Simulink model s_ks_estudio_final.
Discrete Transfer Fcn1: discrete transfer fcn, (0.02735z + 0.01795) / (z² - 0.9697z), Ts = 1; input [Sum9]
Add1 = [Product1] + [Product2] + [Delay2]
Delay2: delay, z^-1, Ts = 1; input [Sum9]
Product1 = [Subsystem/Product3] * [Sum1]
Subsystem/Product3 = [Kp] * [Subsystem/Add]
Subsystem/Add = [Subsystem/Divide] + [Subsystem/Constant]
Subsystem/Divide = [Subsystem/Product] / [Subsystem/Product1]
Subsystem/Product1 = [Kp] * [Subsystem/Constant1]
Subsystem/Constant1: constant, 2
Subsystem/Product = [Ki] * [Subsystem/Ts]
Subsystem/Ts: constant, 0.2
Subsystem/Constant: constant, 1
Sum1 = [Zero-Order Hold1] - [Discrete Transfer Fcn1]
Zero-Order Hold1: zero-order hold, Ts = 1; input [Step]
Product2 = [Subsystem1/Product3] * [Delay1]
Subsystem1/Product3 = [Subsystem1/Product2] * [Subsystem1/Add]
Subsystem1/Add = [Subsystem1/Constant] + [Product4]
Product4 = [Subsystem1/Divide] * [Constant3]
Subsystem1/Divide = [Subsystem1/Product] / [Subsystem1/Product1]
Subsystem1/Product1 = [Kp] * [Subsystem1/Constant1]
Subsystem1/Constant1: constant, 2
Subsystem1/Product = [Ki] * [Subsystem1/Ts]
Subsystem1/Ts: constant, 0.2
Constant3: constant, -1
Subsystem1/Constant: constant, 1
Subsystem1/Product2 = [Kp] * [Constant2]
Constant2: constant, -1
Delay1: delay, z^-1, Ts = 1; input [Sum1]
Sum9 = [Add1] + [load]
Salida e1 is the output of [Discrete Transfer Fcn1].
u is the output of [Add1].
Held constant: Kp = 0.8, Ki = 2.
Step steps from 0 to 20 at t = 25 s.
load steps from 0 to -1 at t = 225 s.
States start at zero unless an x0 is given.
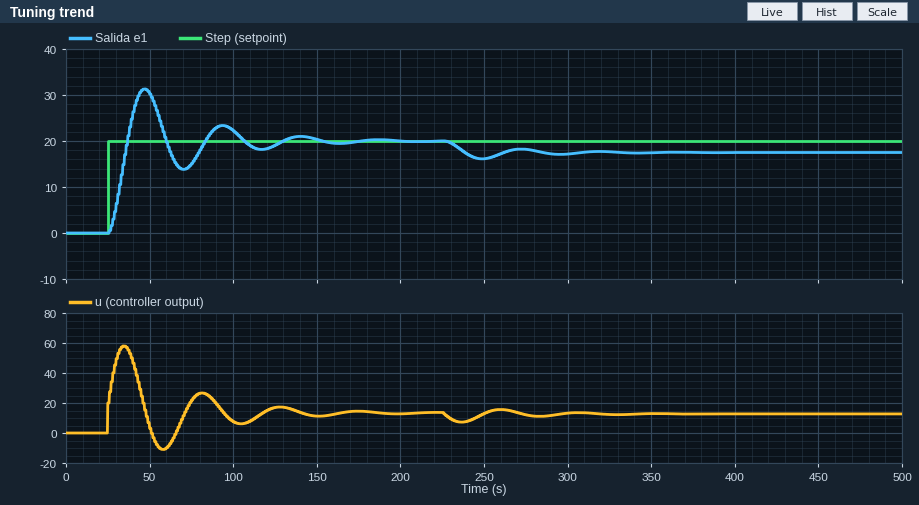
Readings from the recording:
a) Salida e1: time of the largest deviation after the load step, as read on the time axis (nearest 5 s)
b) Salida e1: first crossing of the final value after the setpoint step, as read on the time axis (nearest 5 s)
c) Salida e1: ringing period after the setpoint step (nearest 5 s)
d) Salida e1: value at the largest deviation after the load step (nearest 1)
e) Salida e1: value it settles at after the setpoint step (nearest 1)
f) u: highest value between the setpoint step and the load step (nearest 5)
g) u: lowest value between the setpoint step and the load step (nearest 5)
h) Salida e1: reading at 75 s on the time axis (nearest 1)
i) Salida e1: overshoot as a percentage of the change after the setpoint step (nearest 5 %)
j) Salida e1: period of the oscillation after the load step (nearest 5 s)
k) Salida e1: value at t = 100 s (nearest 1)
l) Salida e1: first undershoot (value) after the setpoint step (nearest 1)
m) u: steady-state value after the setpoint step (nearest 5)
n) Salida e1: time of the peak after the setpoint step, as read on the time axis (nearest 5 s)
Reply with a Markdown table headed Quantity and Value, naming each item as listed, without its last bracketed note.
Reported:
| Quantity | Value |
|---|---|
| Salida e1: time of the largest deviation after the load step, as read on the time axis | 250 s |
| Salida e1: first crossing of the final value after the setpoint step, as read on the time axis | 35 s |
| Salida e1: ringing period after the setpoint step | 45 s |
| Salida e1: value at the largest deviation after the load step | 16 |
| Salida e1: value it settles at after the setpoint step | 20 |
| u: highest value between the setpoint step and the load step | 60 |
| u: lowest value between the setpoint step and the load step | -10 |
| Salida e1: reading at 75 s on the time axis | 15 |
| Salida e1: overshoot as a percentage of the change after the setpoint step | 55 % |
| Salida e1: period of the oscillation after the load step | 45 s |
| Salida e1: value at t = 100 s | 22 |
| Salida e1: first undershoot (value) after the setpoint step | 14 |
| u: steady-state value after the setpoint step | 15 |
| Salida e1: time of the peak after the setpoint step, as read on the time axis | 45 s |
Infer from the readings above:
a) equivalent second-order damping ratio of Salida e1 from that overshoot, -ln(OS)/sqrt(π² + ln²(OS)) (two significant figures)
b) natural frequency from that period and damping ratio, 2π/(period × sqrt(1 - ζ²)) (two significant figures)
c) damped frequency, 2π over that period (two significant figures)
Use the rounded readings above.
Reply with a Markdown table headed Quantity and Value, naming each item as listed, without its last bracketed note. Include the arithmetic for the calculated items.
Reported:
| Quantity | Value |
|---|---|
| equivalent second-order damping ratio of Salida e1 from that overshoot, -ln(OS)/sqrt(π² + ln²(OS)) | ln(0.55) = -0.598; 0.598 / sqrt(9.870 + 0.357) = 0.19 |
| natural frequency from that period and damping ratio, 2π/(period × sqrt(1 - ζ²)) | 2π / (45 × sqrt(1 - 0.19²)) = 0.14 rad/s |
| damped frequency, 2π over that period | 2π / 45 = 0.14 rad/s |
